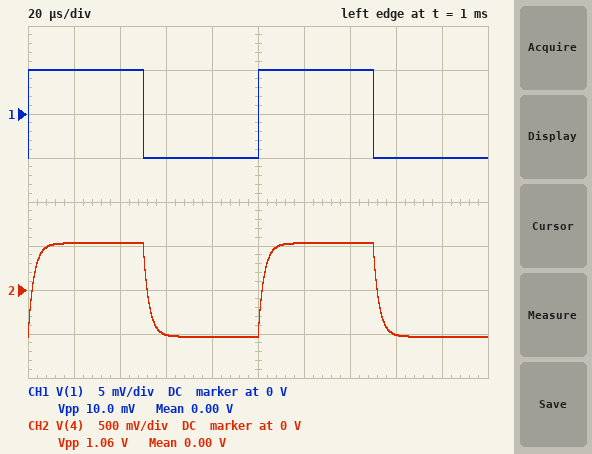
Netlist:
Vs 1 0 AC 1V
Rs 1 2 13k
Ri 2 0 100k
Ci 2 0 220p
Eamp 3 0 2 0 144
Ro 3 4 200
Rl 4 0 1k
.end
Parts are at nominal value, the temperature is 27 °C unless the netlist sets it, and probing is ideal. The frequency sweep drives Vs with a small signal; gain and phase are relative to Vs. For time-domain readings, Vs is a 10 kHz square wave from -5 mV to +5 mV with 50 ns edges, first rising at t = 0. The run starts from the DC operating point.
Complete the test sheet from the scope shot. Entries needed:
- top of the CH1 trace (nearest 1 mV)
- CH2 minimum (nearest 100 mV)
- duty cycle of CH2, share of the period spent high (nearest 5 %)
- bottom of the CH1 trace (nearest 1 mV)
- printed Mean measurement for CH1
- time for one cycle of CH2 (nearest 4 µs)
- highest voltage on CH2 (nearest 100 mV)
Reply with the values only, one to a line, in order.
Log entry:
5 mV
-500 mV
50 %
-5 mV
0.00 V
100 µs
500 mV
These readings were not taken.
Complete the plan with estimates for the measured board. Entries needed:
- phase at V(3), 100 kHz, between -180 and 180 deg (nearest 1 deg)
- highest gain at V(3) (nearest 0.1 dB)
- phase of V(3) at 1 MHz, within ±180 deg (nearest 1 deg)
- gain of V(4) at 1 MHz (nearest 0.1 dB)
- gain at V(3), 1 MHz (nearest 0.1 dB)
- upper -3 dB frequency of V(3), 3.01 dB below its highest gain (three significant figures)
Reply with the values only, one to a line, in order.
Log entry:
-58 deg
42.1 dB
-86 deg
16.5 dB
18.1 dB
62.9 kHz
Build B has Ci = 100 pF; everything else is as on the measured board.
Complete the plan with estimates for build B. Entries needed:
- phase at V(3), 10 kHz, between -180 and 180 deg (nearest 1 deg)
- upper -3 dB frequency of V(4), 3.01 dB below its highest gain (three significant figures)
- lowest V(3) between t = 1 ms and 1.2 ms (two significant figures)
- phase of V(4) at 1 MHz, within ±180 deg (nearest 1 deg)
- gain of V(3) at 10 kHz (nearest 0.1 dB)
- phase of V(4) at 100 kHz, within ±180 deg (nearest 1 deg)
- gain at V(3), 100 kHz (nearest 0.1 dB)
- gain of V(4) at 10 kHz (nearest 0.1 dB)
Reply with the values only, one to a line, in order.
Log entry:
-4 deg
138 kHz
-640 mV
-82 deg
42.1 dB
-36 deg
40.3 dB
40.5 dB
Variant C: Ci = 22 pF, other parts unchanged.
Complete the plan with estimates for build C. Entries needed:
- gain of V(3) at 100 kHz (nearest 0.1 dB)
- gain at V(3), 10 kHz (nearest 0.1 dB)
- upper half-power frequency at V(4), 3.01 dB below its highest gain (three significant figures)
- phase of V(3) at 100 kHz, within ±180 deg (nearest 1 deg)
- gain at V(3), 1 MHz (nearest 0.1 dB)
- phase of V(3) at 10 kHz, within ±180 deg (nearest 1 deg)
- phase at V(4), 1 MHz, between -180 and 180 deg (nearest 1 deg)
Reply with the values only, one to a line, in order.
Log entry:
42.0 dB
42.1 dB
629 kHz
-9 deg
36.6 dB
-1 deg
-58 deg
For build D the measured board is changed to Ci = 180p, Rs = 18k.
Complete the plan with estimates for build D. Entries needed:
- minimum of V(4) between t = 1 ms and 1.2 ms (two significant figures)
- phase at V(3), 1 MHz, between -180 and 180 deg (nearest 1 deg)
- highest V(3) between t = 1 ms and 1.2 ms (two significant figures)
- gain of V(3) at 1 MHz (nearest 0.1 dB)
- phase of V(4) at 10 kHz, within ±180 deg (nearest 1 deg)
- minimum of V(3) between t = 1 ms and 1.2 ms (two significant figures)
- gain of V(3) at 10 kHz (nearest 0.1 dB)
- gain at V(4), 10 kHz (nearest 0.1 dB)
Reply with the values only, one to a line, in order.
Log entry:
-510 mV
-87 deg
610 mV
17.0 dB
-10 deg
-610 mV
41.6 dB
40.0 dB
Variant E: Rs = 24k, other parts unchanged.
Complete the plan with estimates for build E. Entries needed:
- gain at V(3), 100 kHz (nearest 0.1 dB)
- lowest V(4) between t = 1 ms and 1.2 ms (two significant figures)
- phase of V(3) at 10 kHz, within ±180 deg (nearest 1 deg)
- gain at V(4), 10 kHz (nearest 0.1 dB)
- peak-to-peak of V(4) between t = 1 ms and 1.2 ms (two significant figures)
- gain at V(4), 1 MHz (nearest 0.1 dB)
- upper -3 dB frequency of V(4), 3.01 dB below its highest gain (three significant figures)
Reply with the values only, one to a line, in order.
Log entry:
32.2 dB
-480 mV
-15 deg
39.4 dB
970 mV
11.2 dB
37.4 kHz
